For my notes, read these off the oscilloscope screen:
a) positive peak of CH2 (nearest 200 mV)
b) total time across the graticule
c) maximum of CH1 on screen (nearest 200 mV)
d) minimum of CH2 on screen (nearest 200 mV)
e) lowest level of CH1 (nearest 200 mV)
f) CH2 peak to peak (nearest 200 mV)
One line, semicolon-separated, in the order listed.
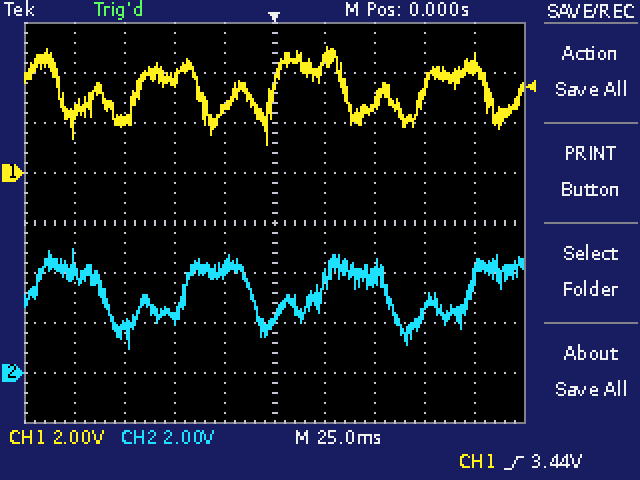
5.0 V; 250 ms; 5.0 V; 1.0 V; 1.2 V; 4.0 V
